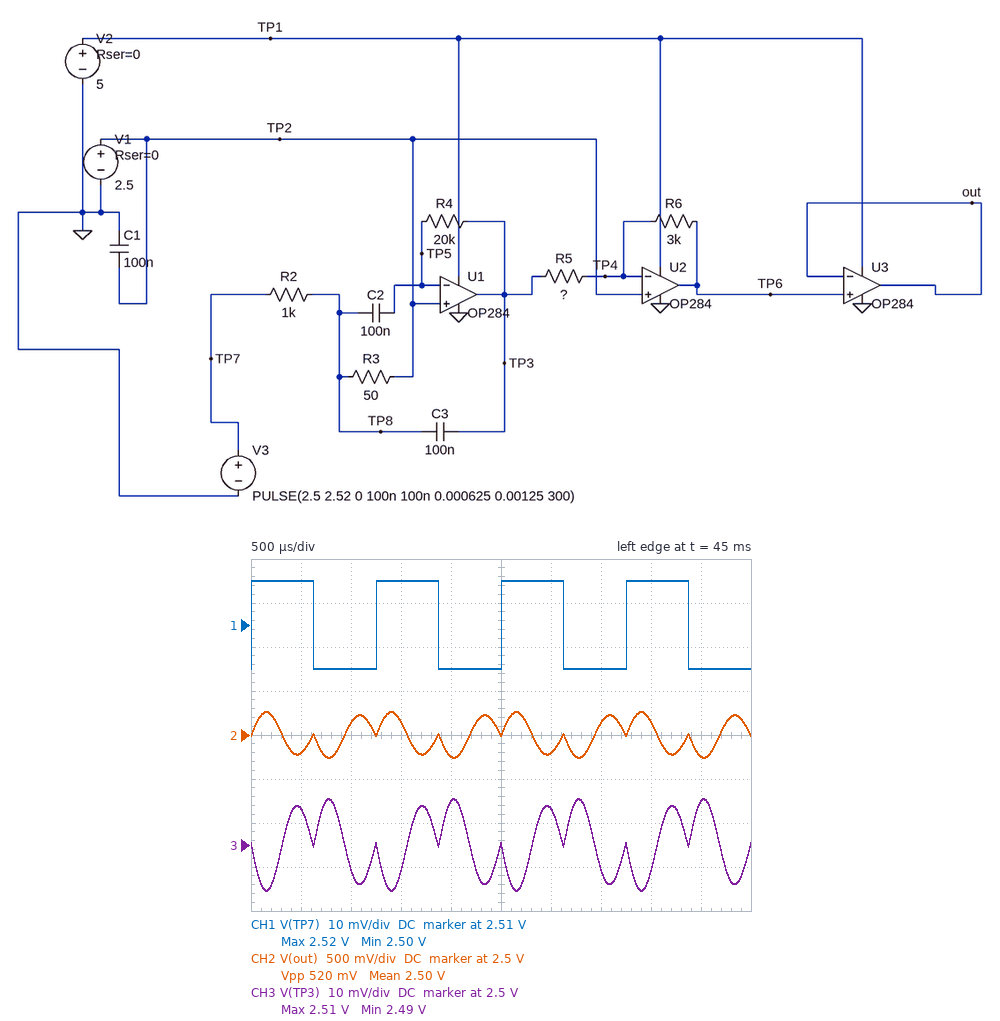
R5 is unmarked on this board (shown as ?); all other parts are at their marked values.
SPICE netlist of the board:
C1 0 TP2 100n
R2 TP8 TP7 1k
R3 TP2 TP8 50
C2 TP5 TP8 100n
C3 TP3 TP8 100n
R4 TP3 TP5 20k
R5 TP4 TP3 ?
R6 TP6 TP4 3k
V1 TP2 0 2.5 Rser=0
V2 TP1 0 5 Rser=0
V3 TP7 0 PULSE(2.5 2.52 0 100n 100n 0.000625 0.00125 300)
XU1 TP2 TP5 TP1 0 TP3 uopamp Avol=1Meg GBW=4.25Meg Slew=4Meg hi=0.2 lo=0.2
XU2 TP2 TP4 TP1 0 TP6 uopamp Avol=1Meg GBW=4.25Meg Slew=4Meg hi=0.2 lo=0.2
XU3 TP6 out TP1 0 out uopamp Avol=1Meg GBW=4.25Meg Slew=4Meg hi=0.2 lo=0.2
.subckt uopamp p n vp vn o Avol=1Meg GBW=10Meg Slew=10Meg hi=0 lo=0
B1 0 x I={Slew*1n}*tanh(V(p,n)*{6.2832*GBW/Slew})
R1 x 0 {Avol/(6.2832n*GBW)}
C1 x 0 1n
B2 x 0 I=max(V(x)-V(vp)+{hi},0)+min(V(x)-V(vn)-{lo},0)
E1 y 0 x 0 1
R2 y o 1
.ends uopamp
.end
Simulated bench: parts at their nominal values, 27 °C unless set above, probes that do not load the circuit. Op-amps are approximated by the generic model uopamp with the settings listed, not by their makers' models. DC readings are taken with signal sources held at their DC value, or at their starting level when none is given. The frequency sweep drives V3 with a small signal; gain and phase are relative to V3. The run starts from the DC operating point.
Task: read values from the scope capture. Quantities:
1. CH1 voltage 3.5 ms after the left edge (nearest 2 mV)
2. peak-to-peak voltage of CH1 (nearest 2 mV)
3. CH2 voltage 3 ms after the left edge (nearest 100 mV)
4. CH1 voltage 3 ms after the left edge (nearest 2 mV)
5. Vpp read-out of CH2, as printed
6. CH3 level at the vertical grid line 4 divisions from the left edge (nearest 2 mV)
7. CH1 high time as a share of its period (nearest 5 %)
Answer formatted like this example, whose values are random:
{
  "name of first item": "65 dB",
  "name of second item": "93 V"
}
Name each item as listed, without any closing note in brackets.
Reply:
{
  "CH1 voltage 3.5 ms after the left edge": "2.500 V",
  "peak-to-peak voltage of CH1": "20 mV",
  "CH2 voltage 3 ms after the left edge": "2.3 V",
  "CH1 voltage 3 ms after the left edge": "2.520 V",
  "Vpp read-out of CH2, as printed": "520 mV",
  "CH3 level at the vertical grid line 4 divisions from the left edge": "2.510 V",
  "CH1 high time as a share of its period": "50 %"
}
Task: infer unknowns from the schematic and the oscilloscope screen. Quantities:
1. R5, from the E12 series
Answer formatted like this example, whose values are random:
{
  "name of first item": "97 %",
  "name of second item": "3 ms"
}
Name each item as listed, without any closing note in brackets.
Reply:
{
  "R5, from the E12 series": "120 Ω"
}
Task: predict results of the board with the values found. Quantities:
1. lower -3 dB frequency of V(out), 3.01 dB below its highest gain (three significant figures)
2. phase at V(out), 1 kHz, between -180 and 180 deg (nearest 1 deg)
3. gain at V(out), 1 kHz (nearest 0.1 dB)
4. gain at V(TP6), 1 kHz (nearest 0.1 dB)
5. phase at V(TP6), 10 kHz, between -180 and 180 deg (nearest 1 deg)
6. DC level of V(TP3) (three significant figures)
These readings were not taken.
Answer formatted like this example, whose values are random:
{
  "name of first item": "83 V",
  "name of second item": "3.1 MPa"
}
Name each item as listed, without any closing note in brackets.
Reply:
{
  "lower -3 dB frequency of V(out), 3.01 dB below its highest gain": "1.55 kHz",
  "phase at V(out), 1 kHz, between -180 and 180 deg": "84 deg",
  "gain at V(out), 1 kHz": "27.6 dB",
  "gain at V(TP6), 1 kHz": "27.6 dB",
  "phase at V(TP6), 10 kHz, between -180 and 180 deg": "-93 deg",
  "DC level of V(TP3)": "2.50 V"
}
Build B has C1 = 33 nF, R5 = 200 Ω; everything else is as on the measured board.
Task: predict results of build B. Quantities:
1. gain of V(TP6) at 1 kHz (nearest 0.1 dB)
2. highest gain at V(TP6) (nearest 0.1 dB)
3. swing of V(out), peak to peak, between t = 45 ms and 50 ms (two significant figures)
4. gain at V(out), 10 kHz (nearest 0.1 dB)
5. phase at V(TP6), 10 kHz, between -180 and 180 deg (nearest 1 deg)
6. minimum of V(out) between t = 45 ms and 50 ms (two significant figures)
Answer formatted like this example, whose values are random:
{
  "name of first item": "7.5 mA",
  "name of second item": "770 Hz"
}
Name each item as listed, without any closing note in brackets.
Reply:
{
  "gain of V(TP6) at 1 kHz": "23.2 dB",
  "highest gain at V(TP6)": "43.5 dB",
  "swing of V(out), peak to peak, between t = 45 ms and 50 ms": "310 mV",
  "gain at V(out), 10 kHz": "7.7 dB",
  "phase at V(TP6), 10 kHz, between -180 and 180 deg": "-91 deg",
  "minimum of V(out) between t = 45 ms and 50 ms": "2.3 V"
}
